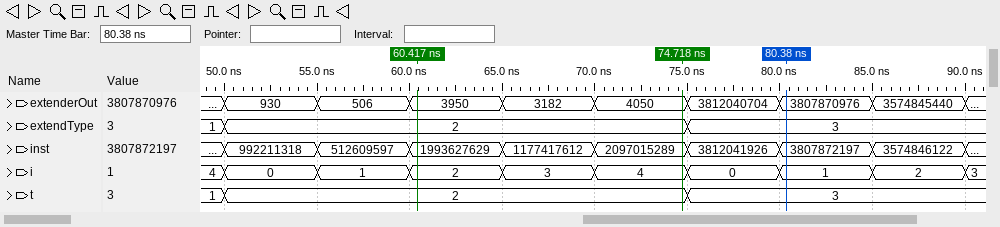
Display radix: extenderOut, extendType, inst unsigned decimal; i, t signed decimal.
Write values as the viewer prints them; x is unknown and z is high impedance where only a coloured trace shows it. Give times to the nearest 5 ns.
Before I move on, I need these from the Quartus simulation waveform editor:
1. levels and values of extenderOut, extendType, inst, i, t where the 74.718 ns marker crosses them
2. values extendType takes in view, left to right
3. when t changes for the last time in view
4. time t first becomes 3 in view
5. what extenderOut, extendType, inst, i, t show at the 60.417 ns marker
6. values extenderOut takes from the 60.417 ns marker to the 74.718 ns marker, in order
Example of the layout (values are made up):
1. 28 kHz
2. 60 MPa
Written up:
1. extenderOut=4050, extendType=2, inst=2097015289, i=4, t=2
2. 1, 2, 3
3. 75 ns
4. 75 ns
5. extenderOut=3950, extendType=2, inst=1993627629, i=2, t=2
6. 3950, 3182, 4050
